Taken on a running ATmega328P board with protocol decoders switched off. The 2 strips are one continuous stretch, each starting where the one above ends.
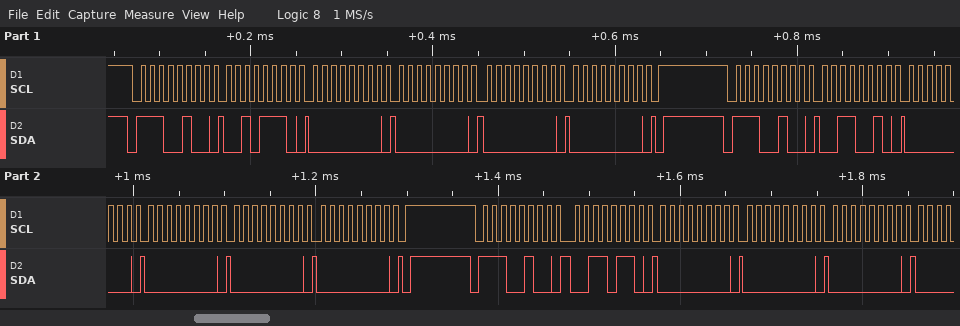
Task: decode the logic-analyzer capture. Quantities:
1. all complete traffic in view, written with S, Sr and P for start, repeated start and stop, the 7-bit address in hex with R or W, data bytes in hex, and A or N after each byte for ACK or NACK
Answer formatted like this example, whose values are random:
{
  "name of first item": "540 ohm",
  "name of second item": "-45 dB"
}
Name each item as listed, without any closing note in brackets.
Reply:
{
  "all complete traffic in view, written with S, Sr and P for start, repeated start and stop, the 7-bit address in hex with R or W, data bytes in hex, and A or N after each byte for ACK or NACK": "S 72W A 2E A 00 A 00 A 00 A 00 A P S 72W A 32 A 00 A 00 A 00 A 00 A P S 72W A 36 A 00 A 00 A 00 A"
}
